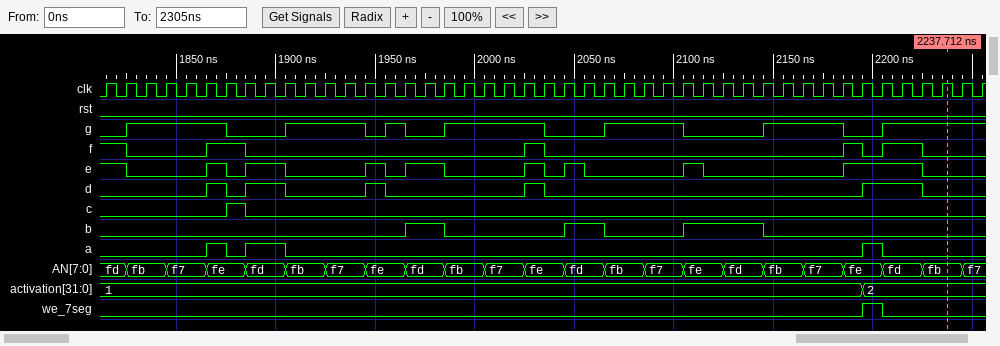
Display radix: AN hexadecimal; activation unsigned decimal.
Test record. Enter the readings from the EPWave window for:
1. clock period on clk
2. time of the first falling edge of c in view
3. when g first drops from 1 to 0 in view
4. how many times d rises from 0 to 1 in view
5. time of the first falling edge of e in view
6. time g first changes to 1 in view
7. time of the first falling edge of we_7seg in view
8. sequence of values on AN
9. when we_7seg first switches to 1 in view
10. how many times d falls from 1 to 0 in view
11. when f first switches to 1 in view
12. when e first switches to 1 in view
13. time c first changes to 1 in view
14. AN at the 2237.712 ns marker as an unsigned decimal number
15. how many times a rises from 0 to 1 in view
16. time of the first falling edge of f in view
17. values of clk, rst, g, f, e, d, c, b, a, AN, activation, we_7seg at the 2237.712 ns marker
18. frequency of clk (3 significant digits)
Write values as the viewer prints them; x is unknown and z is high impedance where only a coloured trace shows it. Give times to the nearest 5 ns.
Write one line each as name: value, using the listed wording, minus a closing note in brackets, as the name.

clock period on clk: 10 ns
time of the first falling edge of c in view: 1885 ns
when g first drops from 1 to 0 in view: 1875 ns
how many times d rises from 0 to 1 in view: 5
time of the first falling edge of e in view: 1825 ns
time g first changes to 1 in view: 1825 ns
time of the first falling edge of we_7seg in view: 2205 ns
sequence of values on AN: fd, fb, f7, fe, fd, fb, f7, fe, fd, fb, f7, fe, fd, fb, f7, fe, fd, fb, f7, fe, fd, fb, f7
when we_7seg first switches to 1 in view: 2195 ns
how many times d falls from 1 to 0 in view: 5
when f first switches to 1 in view: 1865 ns
when e first switches to 1 in view: 1865 ns
time c first changes to 1 in view: 1875 ns
AN at the 2237.712 ns marker as an unsigned decimal number: 251
how many times a rises from 0 to 1 in view: 3
time of the first falling edge of f in view: 1825 ns
values of clk, rst, g, f, e, d, c, b, a, AN, activation, we_7seg at the 2237.712 ns marker: clk=1, rst=0, g=1, f=0, e=0, d=0, c=0, b=0, a=0, AN=fb, activation=2, we_7seg=0
frequency of clk: 100 MHz
